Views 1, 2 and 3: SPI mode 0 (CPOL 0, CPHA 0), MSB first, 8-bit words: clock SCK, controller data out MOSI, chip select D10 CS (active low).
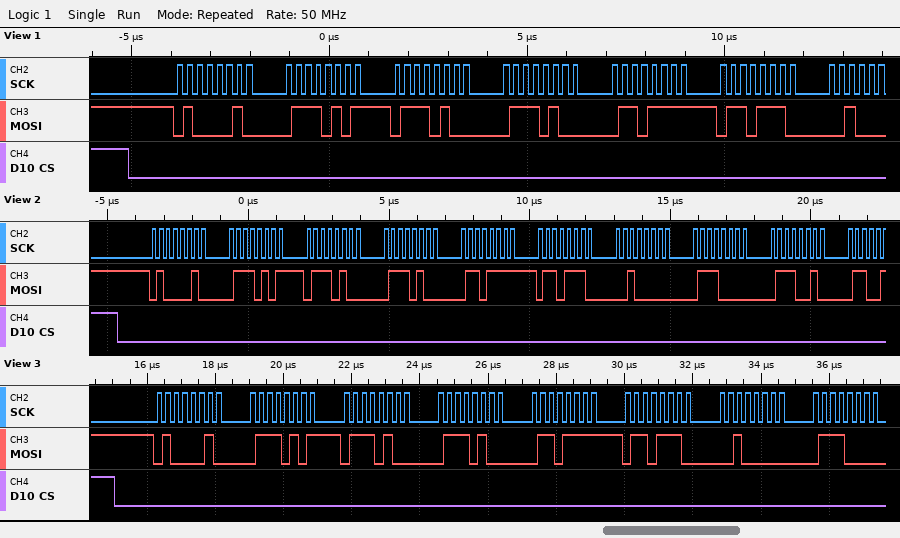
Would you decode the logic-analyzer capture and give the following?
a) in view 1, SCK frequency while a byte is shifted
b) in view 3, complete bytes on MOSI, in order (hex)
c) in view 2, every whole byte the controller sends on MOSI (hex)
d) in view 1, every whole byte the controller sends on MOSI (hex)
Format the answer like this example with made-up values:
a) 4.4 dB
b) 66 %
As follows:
a) 4 MHz
b) 42 75 74 74 6F 6E 20 70
c) 0x42 0x75 0x74 0x74 0x6F 0x6E 0x20 0x70 0x72
d) 0x42 0x75 0x74 0x74 0x6F 0x6E
